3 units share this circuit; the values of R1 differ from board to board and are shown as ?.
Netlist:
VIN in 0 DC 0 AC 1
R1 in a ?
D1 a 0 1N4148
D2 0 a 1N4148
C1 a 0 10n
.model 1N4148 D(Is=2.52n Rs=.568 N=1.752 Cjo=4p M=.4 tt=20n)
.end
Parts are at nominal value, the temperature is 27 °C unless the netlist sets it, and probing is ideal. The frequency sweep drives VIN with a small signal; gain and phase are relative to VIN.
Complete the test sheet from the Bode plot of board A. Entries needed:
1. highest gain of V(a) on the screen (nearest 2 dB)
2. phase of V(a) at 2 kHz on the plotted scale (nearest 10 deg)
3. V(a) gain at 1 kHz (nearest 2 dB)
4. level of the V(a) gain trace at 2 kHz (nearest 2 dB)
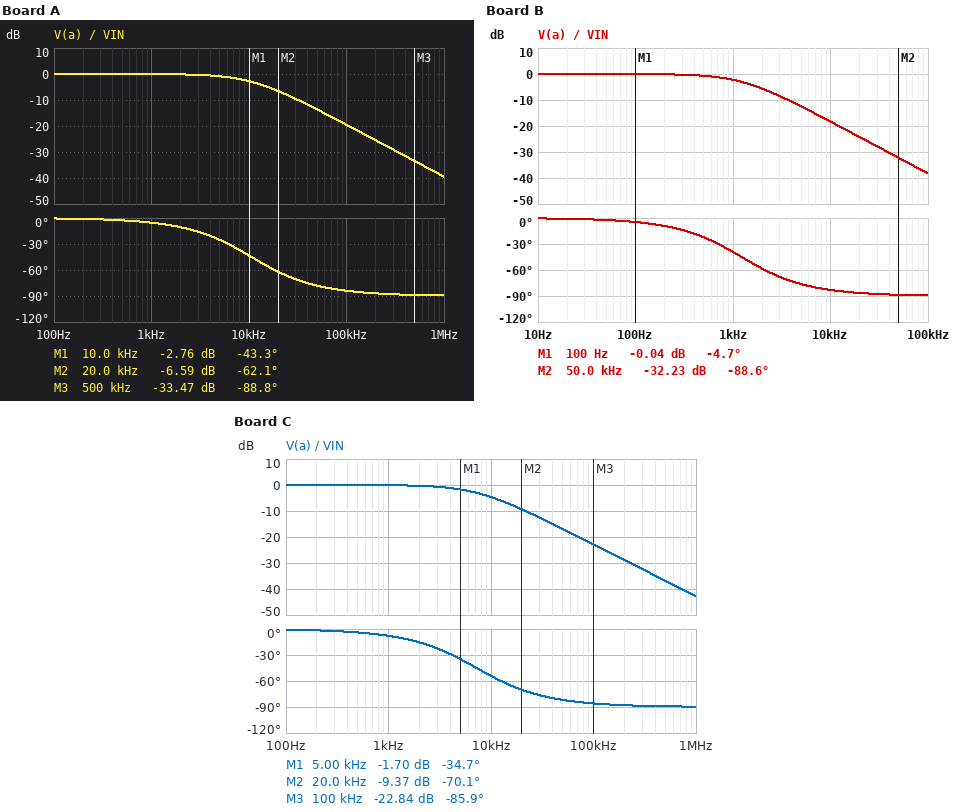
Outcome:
0 dB
-10 deg
0 dB
0 dB
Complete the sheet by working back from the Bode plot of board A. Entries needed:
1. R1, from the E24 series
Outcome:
1.5 kΩ
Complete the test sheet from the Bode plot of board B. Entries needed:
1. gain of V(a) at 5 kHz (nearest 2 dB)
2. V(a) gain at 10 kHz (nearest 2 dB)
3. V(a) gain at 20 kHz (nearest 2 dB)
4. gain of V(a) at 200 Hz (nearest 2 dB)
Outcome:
-12 dB
-18 dB
-24 dB
0 dB
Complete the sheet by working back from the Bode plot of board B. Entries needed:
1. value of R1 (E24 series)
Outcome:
13 kΩ
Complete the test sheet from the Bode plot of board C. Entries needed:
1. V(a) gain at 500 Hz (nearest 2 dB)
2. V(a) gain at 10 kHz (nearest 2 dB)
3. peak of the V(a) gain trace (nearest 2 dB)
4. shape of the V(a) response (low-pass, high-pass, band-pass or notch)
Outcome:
0 dB
-4 dB
0 dB
low-pass
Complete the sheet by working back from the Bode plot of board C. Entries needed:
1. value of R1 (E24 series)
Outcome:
2.2 kΩ
